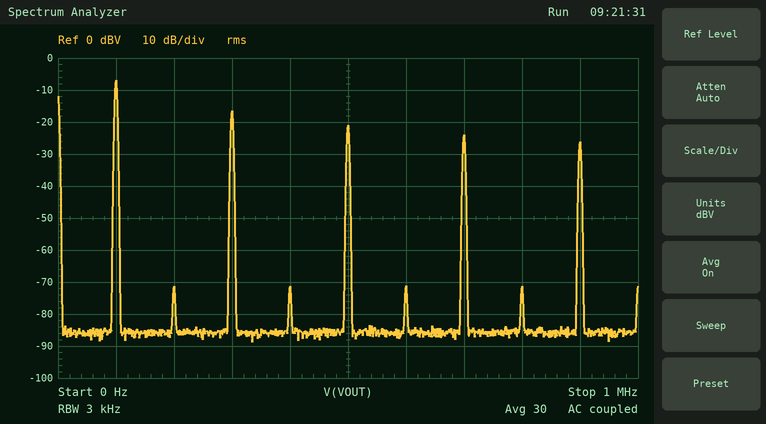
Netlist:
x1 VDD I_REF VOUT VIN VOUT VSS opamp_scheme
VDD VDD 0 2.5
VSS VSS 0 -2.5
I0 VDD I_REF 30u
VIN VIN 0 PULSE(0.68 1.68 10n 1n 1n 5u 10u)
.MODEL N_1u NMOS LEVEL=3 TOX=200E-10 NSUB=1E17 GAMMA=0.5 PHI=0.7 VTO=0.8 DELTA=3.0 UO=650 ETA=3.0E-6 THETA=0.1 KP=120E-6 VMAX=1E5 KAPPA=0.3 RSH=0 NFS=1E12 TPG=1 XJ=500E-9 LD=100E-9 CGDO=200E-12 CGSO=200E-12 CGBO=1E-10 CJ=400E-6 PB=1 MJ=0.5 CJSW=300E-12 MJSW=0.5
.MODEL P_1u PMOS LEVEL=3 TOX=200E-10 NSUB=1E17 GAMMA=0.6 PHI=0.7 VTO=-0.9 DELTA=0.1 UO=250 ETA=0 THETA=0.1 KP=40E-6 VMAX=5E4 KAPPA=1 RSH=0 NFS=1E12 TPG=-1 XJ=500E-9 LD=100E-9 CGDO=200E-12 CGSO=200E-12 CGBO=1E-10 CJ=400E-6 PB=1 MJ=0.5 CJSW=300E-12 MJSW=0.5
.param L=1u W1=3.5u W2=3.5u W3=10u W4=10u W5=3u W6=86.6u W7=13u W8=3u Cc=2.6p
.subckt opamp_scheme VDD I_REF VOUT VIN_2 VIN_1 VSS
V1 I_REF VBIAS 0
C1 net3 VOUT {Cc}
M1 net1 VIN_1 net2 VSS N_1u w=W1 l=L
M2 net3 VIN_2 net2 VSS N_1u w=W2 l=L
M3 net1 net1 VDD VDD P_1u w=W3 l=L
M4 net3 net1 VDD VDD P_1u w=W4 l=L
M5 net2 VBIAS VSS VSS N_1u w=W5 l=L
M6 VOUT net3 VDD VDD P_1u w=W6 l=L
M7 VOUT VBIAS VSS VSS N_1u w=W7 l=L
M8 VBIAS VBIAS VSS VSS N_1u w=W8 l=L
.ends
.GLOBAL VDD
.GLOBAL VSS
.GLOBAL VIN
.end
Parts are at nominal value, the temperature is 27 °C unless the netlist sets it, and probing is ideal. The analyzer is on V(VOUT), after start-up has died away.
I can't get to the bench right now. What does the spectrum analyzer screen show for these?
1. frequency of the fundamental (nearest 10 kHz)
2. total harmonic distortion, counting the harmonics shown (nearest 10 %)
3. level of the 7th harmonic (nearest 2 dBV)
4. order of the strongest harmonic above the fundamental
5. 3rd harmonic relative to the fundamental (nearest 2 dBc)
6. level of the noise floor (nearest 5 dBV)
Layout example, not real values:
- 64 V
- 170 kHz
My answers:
- 100 kHz
- 40 %
- -24 dBV
- 3
- -10 dBc
- -85 dBV
